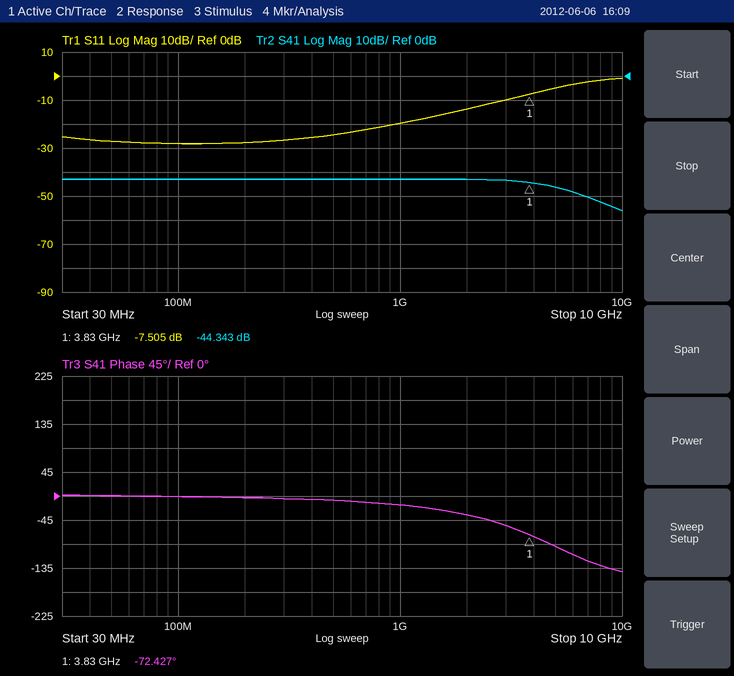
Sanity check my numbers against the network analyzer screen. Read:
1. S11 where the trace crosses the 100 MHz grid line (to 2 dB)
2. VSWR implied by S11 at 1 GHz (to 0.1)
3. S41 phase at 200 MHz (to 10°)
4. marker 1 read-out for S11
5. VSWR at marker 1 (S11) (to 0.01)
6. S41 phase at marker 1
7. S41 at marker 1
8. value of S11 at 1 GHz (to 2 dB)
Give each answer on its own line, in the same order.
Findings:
-28 dB
1.2
0°
-7.505 dB
2.46
-72.427°
-44.343 dB
-20 dB
